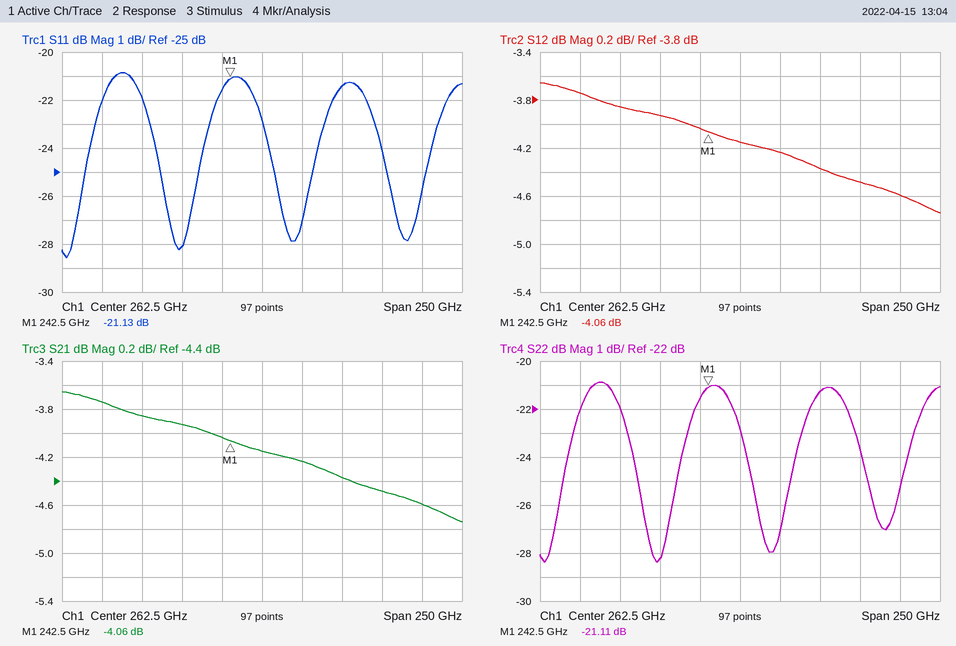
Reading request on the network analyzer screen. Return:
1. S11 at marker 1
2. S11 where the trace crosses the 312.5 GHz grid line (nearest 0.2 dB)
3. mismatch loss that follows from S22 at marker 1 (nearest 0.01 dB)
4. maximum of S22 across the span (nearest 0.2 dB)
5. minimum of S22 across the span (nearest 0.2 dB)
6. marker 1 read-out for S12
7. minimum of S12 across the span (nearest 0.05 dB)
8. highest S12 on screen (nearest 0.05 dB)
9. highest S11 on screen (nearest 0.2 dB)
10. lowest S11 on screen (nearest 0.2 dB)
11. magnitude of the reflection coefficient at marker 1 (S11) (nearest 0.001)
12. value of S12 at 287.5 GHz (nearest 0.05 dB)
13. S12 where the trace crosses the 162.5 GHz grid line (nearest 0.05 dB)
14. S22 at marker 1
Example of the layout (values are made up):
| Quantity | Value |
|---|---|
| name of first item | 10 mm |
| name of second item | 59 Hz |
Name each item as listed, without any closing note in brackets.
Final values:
| Quantity | Value |
|---|---|
| S11 at marker 1 | -21.13 dB |
| S11 where the trace crosses the 312.5 GHz grid line | -21.4 dB |
| mismatch loss that follows from S22 at marker 1 | 0.03 dB |
| maximum of S22 across the span | -20.8 dB |
| minimum of S22 across the span | -28.4 dB |
| marker 1 read-out for S12 | -4.06 dB |
| minimum of S12 across the span | -4.75 dB |
| highest S12 on screen | -3.65 dB |
| highest S11 on screen | -20.8 dB |
| lowest S11 on screen | -28.6 dB |
| magnitude of the reflection coefficient at marker 1 (S11) | 0.088 |
| value of S12 at 287.5 GHz | -4.25 dB |
| S12 where the trace crosses the 162.5 GHz grid line | -3.75 dB |
| S22 at marker 1 | -21.11 dB |
